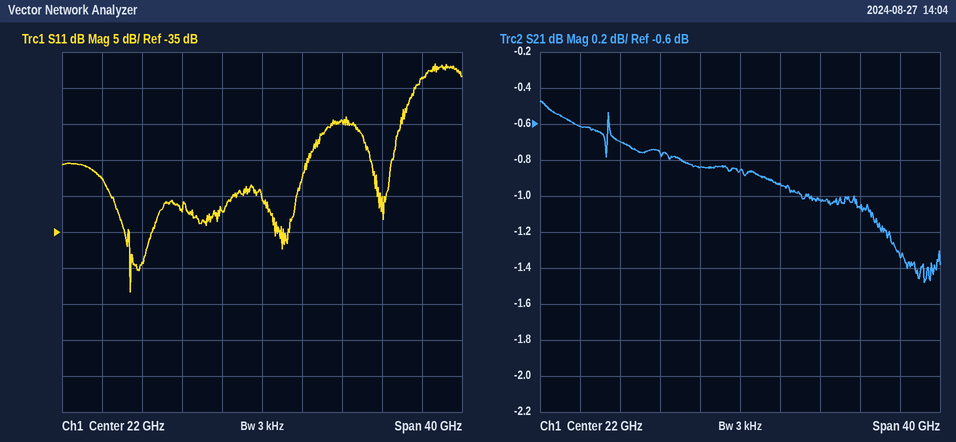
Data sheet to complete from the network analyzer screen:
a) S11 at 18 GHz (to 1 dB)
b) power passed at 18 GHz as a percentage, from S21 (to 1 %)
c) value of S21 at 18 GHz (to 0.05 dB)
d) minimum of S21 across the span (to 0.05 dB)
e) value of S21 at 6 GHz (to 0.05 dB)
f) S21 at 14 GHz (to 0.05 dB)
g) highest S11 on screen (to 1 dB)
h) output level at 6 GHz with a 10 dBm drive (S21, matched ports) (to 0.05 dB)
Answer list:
-32 dB
82 %
-0.85 dB
-1.50 dB
-0.60 dB
-0.75 dB
-12 dB
9.40 dBm
